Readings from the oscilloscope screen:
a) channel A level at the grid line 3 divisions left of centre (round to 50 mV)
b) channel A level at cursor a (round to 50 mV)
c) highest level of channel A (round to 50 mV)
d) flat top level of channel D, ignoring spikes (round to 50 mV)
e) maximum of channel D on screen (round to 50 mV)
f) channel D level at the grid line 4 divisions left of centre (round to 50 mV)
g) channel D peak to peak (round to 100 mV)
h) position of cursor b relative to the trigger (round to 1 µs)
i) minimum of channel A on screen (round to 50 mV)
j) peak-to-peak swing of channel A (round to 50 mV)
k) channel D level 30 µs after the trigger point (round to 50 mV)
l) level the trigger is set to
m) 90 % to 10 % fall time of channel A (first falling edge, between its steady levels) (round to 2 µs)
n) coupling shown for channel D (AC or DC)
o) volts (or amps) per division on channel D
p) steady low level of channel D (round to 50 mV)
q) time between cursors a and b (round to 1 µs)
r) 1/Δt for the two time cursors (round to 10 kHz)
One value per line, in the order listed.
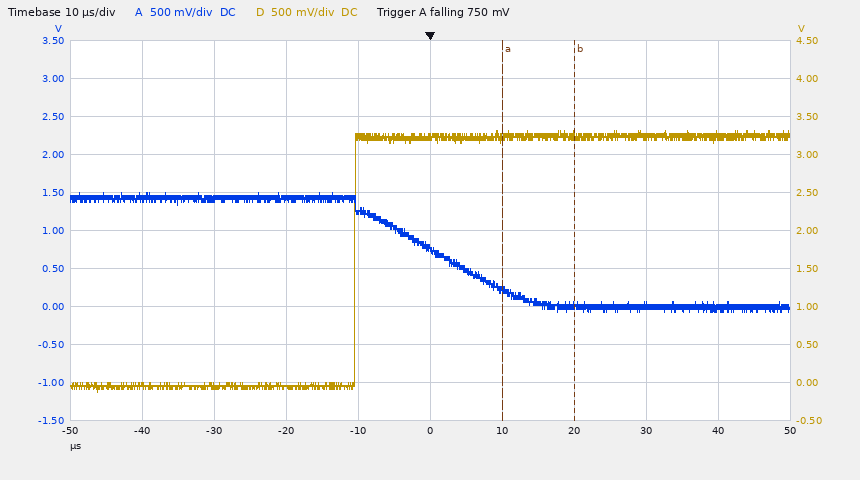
1.40 V
200 mV
1.50 V
3.25 V
3.30 V
-50 mV
3.40 V
+20 µs
-50 mV
1.55 V
3.25 V
750 mV
22 µs
DC
500 mV
-50 mV
10 µs
100 kHz
